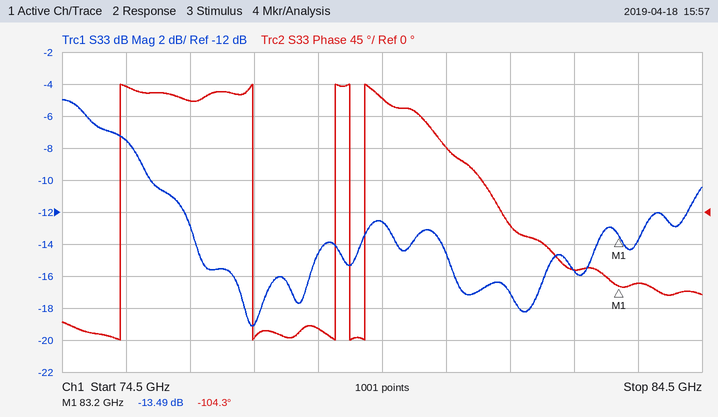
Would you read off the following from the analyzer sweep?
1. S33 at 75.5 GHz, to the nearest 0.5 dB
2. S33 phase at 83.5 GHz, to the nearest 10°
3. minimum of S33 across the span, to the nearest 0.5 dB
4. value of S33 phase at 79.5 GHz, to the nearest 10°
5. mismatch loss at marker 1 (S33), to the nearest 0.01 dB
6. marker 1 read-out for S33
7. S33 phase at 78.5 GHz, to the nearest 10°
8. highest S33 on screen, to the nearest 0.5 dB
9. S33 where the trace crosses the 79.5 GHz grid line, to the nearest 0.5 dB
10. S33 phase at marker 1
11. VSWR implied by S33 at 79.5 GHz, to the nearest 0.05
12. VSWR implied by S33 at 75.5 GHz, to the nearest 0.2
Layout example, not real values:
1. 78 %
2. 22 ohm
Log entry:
1. -7.5 dB
2. -100°
3. -19.0 dB
4. 160°
5. 0.20 dB
6. -13.49 dB
7. -160°
8. -5.0 dB
9. -12.5 dB
10. -104.3°
11. 1.60
12. 2.4
